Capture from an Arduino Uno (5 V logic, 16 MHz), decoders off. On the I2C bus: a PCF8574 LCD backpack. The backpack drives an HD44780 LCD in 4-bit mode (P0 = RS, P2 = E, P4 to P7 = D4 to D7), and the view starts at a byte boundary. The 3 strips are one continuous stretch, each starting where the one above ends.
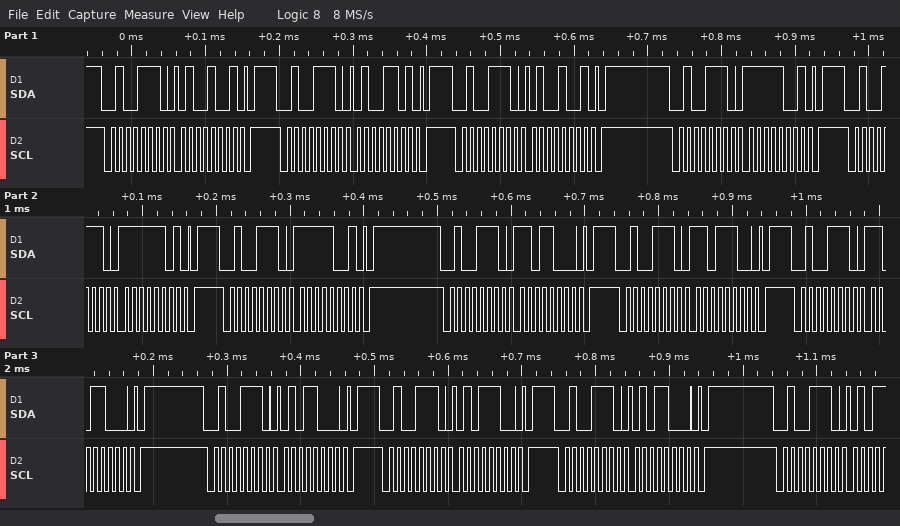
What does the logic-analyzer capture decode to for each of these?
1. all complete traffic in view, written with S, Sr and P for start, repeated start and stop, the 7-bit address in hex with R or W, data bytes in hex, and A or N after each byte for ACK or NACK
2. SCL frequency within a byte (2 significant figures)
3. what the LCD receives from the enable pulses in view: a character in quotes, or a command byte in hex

S 27W A 49 A P S 27W A 4D A P S 27W A 49 A P S 27W A F9 A P S 27W A FD A P S 27W A F9 A P S 27W A D8 A P S 27W A DC A P S 27W A D8 A P S 27W A 58 A P S 27W A 5C A P S 27W A 58 A P S 27W A
100 kHz
'O' 0xD5
